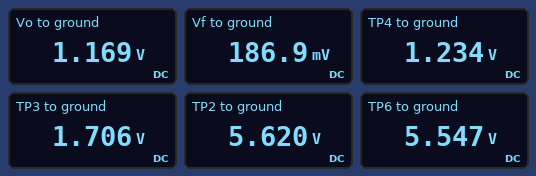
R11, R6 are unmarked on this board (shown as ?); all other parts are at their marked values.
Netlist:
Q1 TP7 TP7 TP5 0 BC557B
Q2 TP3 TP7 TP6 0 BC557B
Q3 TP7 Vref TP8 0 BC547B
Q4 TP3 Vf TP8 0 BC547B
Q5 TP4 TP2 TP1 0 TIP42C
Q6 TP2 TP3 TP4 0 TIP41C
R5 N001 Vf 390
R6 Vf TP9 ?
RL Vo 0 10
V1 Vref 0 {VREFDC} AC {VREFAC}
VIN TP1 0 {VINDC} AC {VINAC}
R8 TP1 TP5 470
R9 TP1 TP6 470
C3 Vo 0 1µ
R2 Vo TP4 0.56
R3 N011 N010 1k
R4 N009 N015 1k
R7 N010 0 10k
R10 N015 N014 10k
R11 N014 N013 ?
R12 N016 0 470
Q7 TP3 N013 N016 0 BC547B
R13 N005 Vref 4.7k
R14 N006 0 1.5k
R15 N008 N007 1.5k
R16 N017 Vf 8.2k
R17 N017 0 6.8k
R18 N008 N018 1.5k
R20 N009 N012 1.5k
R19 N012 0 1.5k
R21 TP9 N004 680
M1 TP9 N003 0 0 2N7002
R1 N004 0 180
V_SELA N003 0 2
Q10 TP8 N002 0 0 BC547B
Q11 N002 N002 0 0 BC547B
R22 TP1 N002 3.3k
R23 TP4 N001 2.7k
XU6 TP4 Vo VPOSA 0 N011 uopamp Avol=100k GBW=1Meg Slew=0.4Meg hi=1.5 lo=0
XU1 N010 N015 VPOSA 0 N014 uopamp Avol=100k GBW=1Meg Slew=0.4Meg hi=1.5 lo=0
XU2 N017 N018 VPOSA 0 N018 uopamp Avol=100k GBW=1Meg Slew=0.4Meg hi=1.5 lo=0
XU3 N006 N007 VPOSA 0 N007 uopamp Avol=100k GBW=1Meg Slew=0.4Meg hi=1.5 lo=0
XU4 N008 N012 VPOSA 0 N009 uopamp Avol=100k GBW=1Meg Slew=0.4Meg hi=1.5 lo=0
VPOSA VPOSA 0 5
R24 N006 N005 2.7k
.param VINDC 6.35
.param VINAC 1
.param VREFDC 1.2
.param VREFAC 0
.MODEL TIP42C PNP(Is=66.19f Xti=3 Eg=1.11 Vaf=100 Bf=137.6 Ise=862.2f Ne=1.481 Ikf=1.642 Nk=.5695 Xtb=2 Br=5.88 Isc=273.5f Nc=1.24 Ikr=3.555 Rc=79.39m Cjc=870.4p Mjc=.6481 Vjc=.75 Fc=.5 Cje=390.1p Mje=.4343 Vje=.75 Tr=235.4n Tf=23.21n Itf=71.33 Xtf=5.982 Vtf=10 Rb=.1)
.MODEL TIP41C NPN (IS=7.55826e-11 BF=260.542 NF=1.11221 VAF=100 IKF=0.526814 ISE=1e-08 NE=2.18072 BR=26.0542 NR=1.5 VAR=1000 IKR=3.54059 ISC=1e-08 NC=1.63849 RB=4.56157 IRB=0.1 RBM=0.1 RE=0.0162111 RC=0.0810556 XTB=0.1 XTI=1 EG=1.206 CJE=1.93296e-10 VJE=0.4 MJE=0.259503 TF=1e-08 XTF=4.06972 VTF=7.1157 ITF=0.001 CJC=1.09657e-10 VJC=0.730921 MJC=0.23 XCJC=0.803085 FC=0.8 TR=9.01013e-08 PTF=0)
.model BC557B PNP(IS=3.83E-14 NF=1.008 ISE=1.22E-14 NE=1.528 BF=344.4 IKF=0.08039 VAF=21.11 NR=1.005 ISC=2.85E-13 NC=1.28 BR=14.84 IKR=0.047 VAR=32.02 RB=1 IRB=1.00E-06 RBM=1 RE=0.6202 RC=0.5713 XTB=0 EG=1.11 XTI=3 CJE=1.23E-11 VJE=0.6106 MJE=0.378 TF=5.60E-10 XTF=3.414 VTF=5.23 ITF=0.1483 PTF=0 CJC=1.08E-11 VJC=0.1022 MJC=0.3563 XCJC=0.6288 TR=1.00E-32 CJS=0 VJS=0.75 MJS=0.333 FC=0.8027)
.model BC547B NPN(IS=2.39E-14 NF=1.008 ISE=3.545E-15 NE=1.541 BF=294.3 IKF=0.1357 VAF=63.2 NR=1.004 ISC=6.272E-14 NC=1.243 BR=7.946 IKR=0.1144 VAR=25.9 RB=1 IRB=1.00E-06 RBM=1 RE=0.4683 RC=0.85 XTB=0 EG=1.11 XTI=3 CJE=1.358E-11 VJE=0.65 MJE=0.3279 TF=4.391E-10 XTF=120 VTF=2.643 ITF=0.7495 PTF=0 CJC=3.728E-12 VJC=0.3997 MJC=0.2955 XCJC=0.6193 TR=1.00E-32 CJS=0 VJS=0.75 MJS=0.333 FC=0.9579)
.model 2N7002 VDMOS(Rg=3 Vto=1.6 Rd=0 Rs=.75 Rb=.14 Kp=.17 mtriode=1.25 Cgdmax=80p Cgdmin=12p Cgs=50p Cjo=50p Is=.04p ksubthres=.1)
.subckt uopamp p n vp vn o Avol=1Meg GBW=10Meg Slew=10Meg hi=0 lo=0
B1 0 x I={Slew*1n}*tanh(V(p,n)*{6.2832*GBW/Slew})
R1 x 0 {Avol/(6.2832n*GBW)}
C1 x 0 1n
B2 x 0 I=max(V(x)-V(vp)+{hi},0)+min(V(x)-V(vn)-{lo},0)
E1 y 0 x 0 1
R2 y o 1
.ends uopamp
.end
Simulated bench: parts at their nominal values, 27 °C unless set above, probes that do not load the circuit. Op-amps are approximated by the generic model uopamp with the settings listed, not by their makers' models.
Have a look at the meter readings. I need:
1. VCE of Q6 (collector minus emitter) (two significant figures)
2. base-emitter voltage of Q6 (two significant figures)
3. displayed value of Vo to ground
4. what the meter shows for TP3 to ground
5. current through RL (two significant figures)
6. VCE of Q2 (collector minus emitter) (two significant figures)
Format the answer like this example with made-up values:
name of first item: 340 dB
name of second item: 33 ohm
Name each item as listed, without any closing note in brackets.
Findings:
VCE of Q6 (collector minus emitter): 4.4 V
base-emitter voltage of Q6: 470 mV
displayed value of Vo to ground: 1.169 V
what the meter shows for TP3 to ground: 1.706 V
current through RL: 120 mA
VCE of Q2 (collector minus emitter): -3.8 V
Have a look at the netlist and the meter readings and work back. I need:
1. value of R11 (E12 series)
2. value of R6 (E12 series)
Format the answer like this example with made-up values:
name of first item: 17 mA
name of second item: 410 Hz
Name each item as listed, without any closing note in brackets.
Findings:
value of R11: 560 Ω
value of R6: 560 Ω
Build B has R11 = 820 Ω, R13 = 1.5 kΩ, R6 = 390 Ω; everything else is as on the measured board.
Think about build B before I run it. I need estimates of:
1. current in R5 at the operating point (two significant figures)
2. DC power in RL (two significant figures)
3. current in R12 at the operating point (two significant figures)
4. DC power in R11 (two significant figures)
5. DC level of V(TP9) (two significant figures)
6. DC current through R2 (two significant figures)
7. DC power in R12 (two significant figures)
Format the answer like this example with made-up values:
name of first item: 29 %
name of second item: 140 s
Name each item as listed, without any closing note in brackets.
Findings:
current in R5 at the operating point: 300 µA
DC power in RL: 100 mW
current in R12 at the operating point: 3.2 mA
DC power in R11: 2.0 mW
DC level of V(TP9): 3.7 mV
DC current through R2: 100 mA
DC power in R12: 4.9 mW
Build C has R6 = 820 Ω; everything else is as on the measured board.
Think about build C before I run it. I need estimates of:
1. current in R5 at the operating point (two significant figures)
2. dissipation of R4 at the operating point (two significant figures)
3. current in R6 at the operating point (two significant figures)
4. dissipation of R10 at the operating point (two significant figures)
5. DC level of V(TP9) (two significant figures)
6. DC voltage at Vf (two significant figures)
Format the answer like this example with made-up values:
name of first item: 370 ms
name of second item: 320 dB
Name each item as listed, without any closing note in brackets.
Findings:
current in R5 at the operating point: 320 µA
dissipation of R4 at the operating point: 84 µW
current in R6 at the operating point: 300 µA
dissipation of R10 at the operating point: 840 µW
DC level of V(TP9): 3.7 mV
DC voltage at Vf: 250 mV
